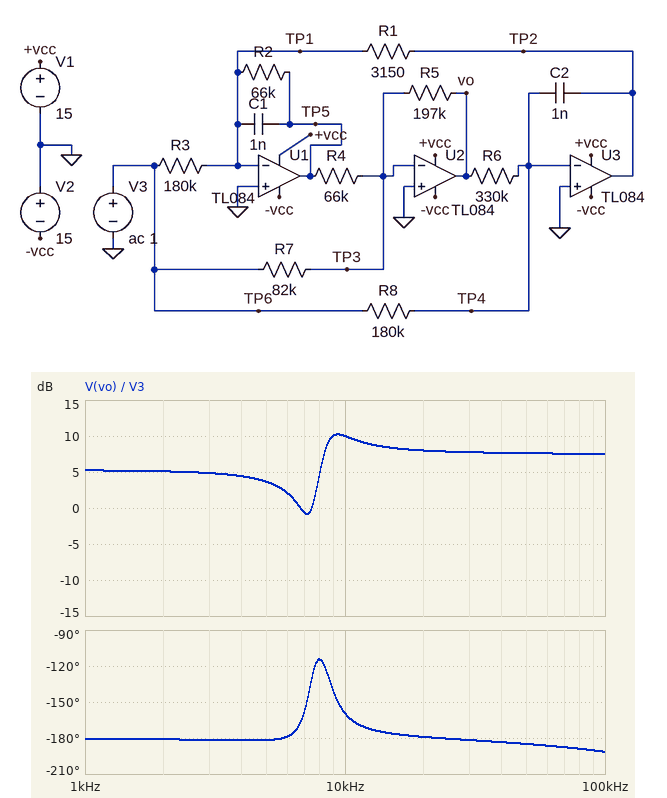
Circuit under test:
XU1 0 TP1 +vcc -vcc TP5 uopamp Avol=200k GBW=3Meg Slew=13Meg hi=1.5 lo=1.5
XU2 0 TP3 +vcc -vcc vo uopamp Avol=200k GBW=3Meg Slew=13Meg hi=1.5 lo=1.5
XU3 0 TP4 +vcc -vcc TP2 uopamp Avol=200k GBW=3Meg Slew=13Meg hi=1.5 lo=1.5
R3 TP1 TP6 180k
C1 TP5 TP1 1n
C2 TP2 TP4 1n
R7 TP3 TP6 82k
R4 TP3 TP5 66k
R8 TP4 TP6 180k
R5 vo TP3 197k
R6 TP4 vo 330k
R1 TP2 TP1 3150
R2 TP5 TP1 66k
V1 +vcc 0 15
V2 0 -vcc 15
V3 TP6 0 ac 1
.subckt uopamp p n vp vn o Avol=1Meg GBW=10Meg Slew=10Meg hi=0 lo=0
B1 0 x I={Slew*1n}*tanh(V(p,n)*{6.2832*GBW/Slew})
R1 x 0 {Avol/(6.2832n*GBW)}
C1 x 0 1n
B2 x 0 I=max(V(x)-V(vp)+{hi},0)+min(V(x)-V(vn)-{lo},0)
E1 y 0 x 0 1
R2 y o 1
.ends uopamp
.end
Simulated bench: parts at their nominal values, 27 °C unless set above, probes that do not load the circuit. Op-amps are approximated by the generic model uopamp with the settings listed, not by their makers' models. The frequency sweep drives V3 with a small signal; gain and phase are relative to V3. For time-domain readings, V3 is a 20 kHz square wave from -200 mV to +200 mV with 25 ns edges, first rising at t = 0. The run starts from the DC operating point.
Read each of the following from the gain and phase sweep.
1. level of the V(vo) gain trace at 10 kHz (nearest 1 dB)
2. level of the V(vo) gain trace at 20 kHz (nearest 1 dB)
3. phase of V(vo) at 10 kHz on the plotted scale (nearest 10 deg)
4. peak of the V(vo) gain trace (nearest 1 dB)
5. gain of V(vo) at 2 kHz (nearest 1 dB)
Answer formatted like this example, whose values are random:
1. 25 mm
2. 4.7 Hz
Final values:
1. 10 dB
2. 8 dB
3. -160 deg
4. 10 dB
5. 5 dB
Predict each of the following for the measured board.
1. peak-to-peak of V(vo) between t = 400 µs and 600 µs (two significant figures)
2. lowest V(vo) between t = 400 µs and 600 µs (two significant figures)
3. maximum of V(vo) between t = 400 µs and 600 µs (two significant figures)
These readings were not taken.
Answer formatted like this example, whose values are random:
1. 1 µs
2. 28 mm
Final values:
1. 1.1 V
2. -530 mV
3. 530 mV
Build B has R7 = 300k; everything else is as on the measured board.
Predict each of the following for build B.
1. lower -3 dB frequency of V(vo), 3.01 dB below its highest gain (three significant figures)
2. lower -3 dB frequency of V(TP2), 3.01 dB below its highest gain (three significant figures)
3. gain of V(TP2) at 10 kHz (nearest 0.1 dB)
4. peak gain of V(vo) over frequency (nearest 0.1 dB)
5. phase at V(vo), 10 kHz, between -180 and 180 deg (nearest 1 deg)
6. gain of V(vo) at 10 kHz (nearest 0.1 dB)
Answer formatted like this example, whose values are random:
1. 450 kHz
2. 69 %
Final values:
1. 6.67 kHz
2. 7.35 kHz
3. -15.3 dB
4. 13.4 dB
5. 27 deg
6. 5.3 dB
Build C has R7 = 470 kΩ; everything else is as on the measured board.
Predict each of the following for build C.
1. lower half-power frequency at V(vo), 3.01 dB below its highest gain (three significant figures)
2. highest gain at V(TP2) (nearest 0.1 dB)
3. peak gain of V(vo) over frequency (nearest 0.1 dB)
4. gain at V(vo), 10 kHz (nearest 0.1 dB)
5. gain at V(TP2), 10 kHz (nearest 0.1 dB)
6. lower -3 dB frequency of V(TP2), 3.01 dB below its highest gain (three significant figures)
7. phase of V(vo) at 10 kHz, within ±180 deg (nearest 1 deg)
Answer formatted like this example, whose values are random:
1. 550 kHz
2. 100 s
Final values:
1. 6.89 kHz
2. -9.3 dB
3. 14.9 dB
4. 8.0 dB
5. -13.8 dB
6. 7.36 kHz
7. 26 deg
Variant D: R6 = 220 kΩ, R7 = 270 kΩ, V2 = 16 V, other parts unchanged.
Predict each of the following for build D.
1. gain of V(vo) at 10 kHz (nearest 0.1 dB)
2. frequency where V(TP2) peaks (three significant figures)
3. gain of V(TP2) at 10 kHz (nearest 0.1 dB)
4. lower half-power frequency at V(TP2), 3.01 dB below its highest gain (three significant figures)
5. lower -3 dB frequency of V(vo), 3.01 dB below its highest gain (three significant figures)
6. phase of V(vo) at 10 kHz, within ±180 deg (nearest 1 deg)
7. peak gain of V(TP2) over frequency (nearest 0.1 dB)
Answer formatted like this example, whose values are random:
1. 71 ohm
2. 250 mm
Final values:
1. 8.3 dB
2. 10.3 kHz
3. -14.1 dB
4. 9.26 kHz
5. 8.09 kHz
6. 98 deg
7. -13.8 dB
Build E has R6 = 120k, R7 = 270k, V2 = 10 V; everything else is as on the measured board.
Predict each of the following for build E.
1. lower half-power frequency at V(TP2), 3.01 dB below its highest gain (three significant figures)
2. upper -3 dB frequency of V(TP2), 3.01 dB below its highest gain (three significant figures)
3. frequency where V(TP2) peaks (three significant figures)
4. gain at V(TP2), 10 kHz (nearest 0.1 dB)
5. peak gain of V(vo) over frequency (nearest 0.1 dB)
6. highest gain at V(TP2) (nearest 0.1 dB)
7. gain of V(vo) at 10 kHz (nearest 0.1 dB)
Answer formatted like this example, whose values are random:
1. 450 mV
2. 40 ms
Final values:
1. 12.9 kHz
2. 14.9 kHz
3. 13.9 kHz
4. -29.7 dB
5. -1.0 dB
6. -18.6 dB
7. -4.5 dB
